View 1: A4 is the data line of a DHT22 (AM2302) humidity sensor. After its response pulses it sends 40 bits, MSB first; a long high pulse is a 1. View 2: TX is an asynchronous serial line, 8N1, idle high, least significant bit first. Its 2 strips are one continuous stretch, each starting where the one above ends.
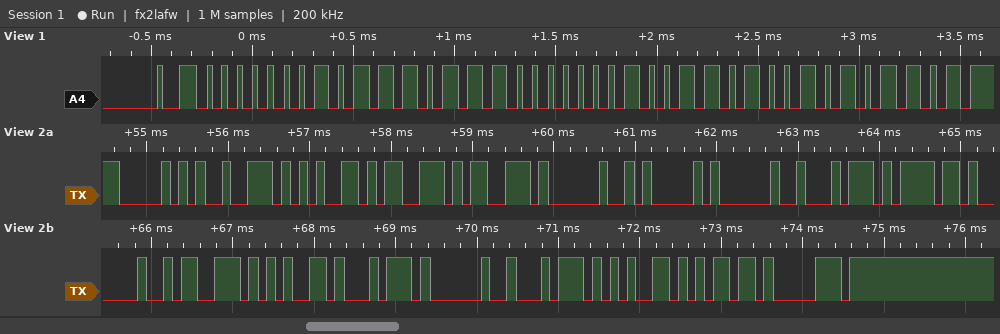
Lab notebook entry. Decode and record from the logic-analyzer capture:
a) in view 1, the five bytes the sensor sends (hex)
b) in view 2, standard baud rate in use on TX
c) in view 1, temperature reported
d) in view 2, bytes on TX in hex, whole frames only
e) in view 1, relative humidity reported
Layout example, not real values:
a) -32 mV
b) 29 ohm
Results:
a) 01 77 01 34 AD
b) 9600 baud
c) 30.8 °C
d) 50 72 65 73 73 20 41 20 74 6F 20 73 65 74 20 74 65 6D 70
e) 37.5 %
